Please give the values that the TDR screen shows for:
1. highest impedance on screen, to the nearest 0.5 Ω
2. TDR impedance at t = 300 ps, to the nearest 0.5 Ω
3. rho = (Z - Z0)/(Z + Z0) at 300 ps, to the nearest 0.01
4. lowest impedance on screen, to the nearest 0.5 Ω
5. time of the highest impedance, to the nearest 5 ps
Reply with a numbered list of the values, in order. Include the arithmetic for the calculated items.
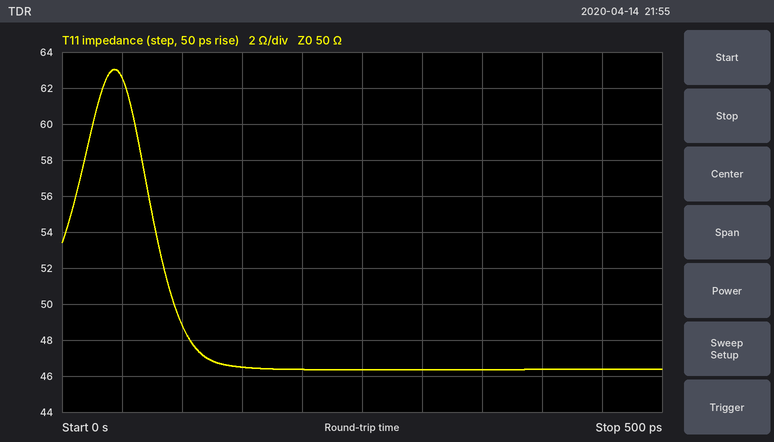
1. 63.0 Ω
2. 46.5 Ω
3. (46.5 − 50)/(46.5 + 50) ≈ -0.04
4. 46.5 Ω
5. 45 ps
